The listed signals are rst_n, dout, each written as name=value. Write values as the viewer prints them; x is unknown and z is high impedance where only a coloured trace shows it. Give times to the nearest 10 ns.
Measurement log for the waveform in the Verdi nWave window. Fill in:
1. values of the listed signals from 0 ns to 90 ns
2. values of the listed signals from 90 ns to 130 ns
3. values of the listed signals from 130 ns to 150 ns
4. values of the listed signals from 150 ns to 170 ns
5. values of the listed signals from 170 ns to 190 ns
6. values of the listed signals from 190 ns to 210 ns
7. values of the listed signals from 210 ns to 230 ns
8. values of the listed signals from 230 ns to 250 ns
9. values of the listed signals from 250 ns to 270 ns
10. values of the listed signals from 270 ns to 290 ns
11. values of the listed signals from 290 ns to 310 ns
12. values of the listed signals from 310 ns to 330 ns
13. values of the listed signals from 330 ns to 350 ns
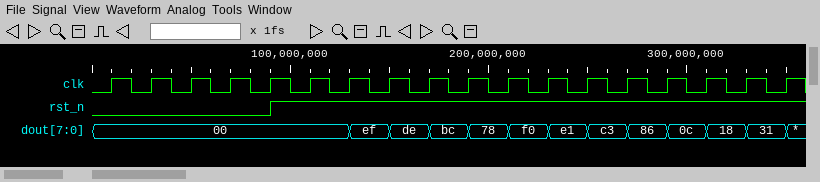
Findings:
rst_n=0, dout=00
rst_n=1, dout=00
rst_n=1, dout=ef
rst_n=1, dout=de
rst_n=1, dout=bc
rst_n=1, dout=78
rst_n=1, dout=f0
rst_n=1, dout=e1
rst_n=1, dout=c3
rst_n=1, dout=86
rst_n=1, dout=0c
rst_n=1, dout=18
rst_n=1, dout=31
